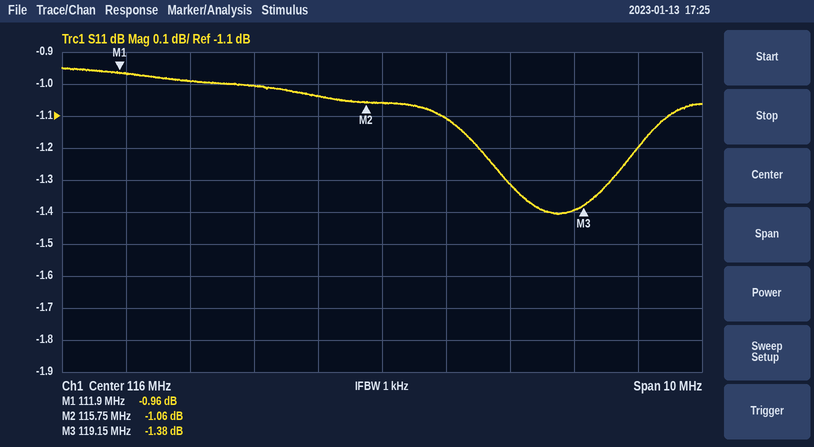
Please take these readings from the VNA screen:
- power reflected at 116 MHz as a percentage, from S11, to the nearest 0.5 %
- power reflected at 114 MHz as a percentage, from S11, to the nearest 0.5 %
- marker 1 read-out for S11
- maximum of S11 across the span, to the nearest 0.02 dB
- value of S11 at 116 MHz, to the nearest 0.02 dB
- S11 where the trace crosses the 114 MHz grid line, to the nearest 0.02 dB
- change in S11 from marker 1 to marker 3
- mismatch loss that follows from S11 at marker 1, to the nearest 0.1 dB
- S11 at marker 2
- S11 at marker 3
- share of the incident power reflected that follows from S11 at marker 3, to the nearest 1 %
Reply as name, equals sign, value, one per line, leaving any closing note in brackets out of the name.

power reflected at 116 MHz as a percentage, from S11, to the nearest 0.5 % = 78.5 %
power reflected at 114 MHz as a percentage, from S11, to the nearest 0.5 % = 79.5 %
marker 1 read-out for S11 = -0.96 dB
maximum of S11 across the span, to the nearest 0.02 dB = -0.94 dB
value of S11 at 116 MHz, to the nearest 0.02 dB = -1.06 dB
S11 where the trace crosses the 114 MHz grid line, to the nearest 0.02 dB = -1.00 dB
change in S11 from marker 1 to marker 3 = -0.42 dB
mismatch loss that follows from S11 at marker 1, to the nearest 0.1 dB = 7.0 dB
S11 at marker 2 = -1.06 dB
S11 at marker 3 = -1.38 dB
share of the incident power reflected that follows from S11 at marker 3, to the nearest 1 % = 73 %
